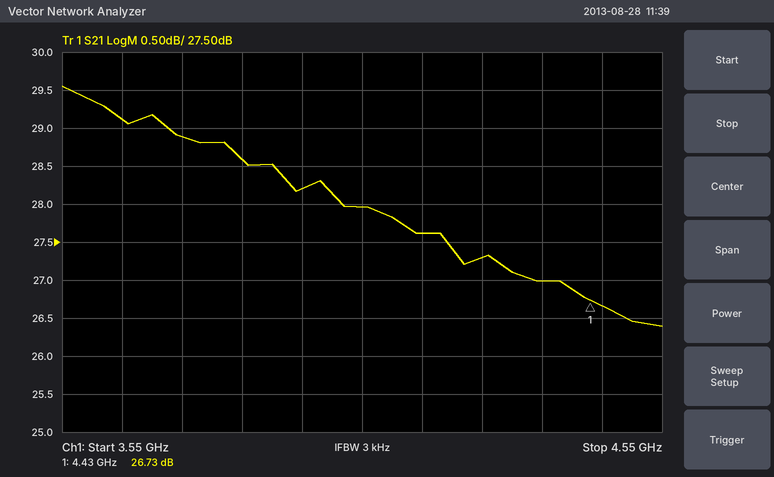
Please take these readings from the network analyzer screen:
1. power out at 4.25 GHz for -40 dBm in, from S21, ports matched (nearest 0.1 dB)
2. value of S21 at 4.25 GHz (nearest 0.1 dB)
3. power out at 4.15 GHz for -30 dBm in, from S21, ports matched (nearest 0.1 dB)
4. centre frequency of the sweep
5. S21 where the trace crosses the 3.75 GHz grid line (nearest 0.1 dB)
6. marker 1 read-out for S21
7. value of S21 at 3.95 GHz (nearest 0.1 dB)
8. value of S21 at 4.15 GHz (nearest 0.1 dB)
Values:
-12.7 dBm
27.3 dB
-2.4 dBm
4.05 GHz
28.9 dB
26.73 dB
28.2 dB
27.6 dB
